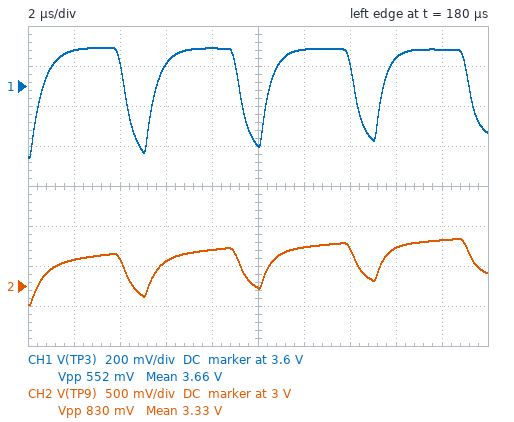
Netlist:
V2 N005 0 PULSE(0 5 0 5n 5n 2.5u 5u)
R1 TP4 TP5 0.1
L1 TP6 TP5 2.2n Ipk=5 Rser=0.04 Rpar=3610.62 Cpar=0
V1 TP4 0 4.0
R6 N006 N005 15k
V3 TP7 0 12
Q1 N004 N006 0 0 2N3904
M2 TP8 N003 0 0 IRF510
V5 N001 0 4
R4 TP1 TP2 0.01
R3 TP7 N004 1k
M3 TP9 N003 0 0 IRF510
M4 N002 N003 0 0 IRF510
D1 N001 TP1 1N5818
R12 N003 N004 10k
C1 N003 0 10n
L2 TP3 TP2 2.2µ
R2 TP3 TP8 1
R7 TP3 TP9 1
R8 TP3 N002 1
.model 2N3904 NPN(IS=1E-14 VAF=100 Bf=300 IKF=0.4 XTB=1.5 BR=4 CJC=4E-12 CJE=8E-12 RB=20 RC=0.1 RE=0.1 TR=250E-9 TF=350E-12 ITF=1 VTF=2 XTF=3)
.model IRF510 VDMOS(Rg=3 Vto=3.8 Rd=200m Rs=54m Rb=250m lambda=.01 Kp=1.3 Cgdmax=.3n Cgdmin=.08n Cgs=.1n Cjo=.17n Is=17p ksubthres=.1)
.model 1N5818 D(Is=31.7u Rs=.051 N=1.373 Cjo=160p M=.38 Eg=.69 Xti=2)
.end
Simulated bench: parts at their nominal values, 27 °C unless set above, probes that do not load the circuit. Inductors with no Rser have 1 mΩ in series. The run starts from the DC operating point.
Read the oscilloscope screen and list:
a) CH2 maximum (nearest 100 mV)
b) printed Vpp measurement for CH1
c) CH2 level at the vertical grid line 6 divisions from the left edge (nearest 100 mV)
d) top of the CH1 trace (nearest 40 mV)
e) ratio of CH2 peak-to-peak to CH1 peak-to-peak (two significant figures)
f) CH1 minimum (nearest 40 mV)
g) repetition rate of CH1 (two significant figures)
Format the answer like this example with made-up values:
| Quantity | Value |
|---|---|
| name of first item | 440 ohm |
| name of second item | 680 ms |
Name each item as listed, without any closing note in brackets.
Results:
| Quantity | Value |
|---|---|
| CH2 maximum | 3.6 V |
| printed Vpp measurement for CH1 | 552 mV |
| CH2 level at the vertical grid line 6 divisions from the left edge | 3.5 V |
| top of the CH1 trace | 3.80 V |
| ratio of CH2 peak-to-peak to CH1 peak-to-peak | 1.5 |
| CH1 minimum | 3.24 V |
| repetition rate of CH1 | 200 kHz |
